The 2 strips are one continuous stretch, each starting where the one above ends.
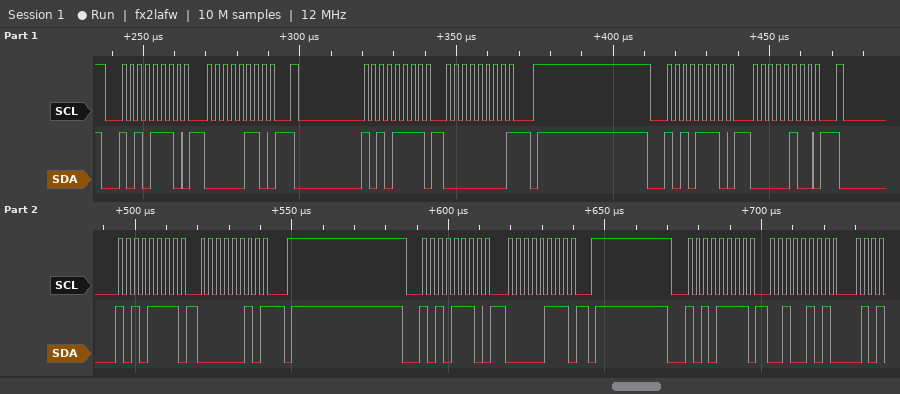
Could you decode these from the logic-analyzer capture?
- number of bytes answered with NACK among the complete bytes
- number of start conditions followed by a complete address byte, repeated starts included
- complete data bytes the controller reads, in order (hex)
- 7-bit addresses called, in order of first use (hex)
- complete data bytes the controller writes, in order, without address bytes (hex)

2
6
00 02 25
0x57
06 04 07
